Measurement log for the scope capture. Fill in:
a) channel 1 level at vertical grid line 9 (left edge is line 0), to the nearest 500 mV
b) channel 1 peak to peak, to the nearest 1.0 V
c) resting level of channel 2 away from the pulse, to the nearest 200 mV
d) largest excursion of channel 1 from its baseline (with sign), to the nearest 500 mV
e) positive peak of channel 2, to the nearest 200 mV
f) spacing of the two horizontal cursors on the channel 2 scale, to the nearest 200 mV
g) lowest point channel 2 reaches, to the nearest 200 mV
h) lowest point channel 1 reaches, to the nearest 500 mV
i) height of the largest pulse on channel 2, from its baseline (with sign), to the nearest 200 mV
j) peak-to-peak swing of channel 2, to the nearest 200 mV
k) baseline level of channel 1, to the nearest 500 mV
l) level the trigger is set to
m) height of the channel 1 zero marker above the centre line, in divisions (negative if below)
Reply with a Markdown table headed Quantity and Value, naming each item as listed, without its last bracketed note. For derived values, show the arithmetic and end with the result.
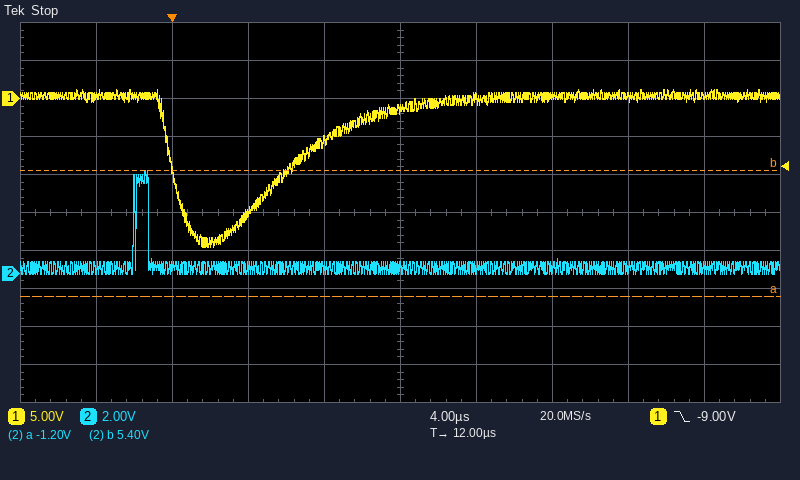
| Quantity | Value |
|---|---|
| channel 1 level at vertical grid line 9 (left edge is line 0), to the nearest 500 mV | 500 mV |
| channel 1 peak to peak, to the nearest 1.0 V | 21.0 V |
| resting level of channel 2 away from the pulse, to the nearest 200 mV | 400 mV |
| largest excursion of channel 1 from its baseline (with sign), to the nearest 500 mV | -19.5 V − (500 mV) = -20.0 V |
| positive peak of channel 2, to the nearest 200 mV | 5.4 V |
| spacing of the two horizontal cursors on the channel 2 scale, to the nearest 200 mV | 6.6 V |
| lowest point channel 2 reaches, to the nearest 200 mV | 0.0 V |
| lowest point channel 1 reaches, to the nearest 500 mV | -19.5 V |
| height of the largest pulse on channel 2, from its baseline (with sign), to the nearest 200 mV | 5.4 V − (400 mV) = +5.0 V |
| peak-to-peak swing of channel 2, to the nearest 200 mV | 5.4 V − (0.0 V) = 5.4 V |
| baseline level of channel 1, to the nearest 500 mV | 500 mV |
| level the trigger is set to | -9.00 V |
| height of the channel 1 zero marker above the centre line, in divisions | +3.0 div |
